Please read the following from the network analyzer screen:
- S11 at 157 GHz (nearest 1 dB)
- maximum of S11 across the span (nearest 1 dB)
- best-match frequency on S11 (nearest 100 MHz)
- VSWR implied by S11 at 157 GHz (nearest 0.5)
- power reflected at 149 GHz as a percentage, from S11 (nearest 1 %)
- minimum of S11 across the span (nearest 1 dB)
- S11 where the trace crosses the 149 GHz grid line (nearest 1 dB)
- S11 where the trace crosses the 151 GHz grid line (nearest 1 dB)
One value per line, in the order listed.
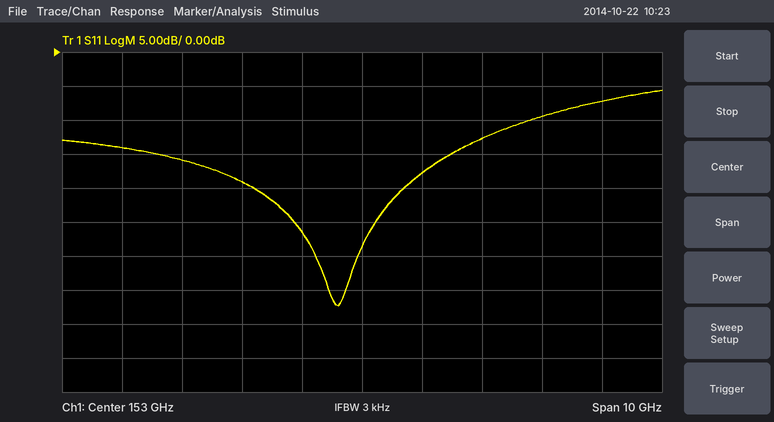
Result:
-7 dB
-6 dB
152.6 GHz
2.5
4 %
-37 dB
-14 dB
-19 dB
